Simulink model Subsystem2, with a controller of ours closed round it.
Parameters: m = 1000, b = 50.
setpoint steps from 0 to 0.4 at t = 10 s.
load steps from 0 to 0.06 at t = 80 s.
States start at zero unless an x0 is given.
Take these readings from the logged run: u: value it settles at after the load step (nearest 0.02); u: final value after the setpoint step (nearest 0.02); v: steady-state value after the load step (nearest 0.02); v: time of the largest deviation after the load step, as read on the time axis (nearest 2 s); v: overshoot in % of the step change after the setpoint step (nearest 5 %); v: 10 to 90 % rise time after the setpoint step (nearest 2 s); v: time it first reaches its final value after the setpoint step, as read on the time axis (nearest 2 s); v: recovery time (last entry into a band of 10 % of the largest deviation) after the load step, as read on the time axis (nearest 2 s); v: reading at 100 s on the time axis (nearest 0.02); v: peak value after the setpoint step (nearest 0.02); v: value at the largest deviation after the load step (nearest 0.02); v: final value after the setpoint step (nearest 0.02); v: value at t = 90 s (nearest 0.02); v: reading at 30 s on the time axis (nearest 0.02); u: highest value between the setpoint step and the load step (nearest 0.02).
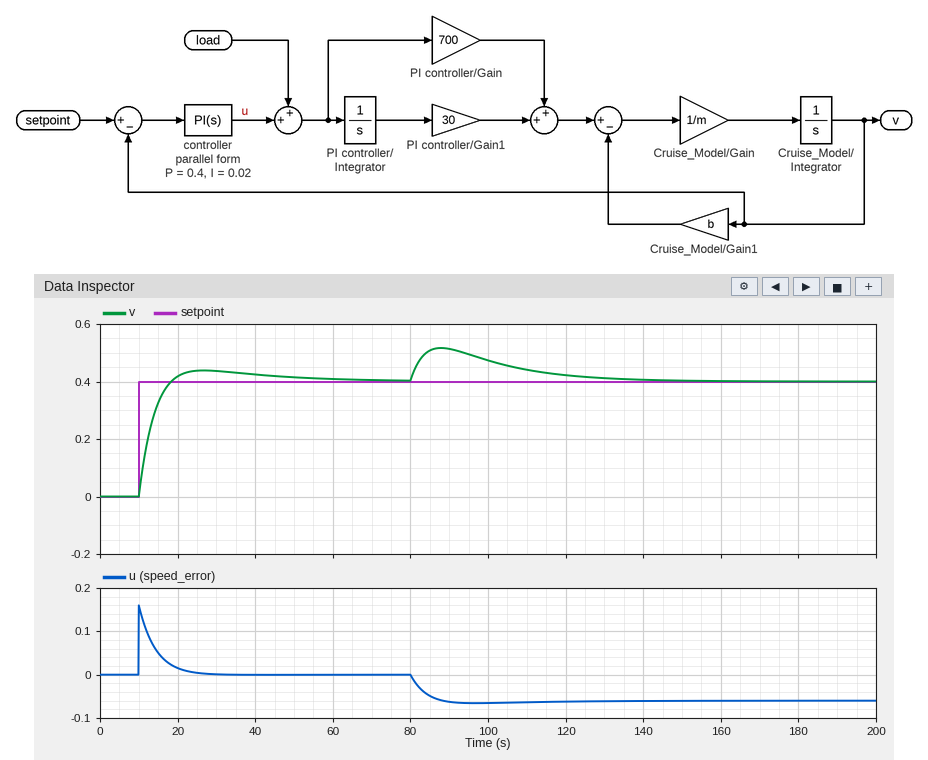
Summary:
-0.06
0.00
0.40
88 s
10 %
6 s
18 s
130 s
0.48
0.44
0.52
0.40
0.52
0.44
0.16
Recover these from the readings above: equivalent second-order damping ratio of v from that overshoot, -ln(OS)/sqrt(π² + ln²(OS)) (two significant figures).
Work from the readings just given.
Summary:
0.59
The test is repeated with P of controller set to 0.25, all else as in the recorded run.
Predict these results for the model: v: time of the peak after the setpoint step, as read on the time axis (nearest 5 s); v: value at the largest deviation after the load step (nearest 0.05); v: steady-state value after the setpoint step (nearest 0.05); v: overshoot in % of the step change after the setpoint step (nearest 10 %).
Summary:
30 s
0.55
0.40
20 %
